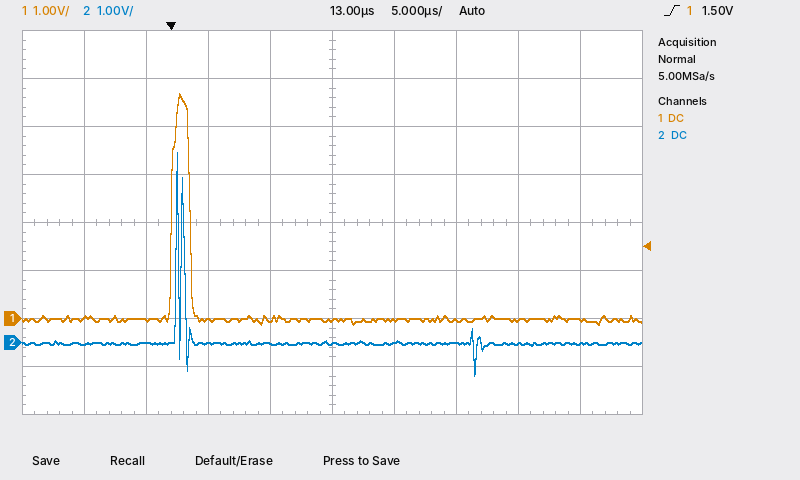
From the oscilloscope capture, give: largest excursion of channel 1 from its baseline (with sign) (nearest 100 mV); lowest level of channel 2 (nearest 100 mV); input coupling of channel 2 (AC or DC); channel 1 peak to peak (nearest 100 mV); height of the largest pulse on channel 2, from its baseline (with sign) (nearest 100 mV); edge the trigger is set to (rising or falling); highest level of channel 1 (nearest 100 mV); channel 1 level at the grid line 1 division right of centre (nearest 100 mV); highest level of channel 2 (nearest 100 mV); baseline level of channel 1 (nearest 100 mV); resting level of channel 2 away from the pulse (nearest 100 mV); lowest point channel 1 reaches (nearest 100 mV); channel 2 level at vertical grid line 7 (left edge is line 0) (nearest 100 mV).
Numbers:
+4.7 V
-700 mV
DC
4.8 V
+4.0 V
rising
4.7 V
0.0 V
4.0 V
0.0 V
0.0 V
-100 mV
0.0 V
